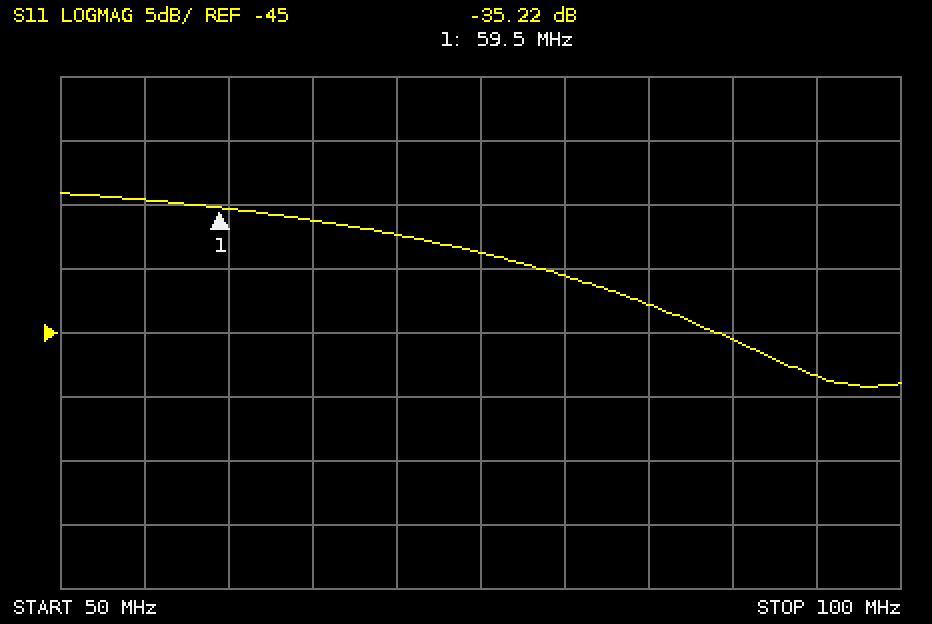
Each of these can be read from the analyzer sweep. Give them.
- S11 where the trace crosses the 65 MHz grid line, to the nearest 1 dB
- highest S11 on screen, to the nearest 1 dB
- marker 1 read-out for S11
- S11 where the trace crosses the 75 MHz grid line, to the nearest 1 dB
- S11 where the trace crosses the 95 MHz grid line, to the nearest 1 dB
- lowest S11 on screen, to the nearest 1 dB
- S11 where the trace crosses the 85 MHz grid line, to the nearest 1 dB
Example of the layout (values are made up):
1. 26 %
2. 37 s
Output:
1. -36 dB
2. -34 dB
3. -35.22 dB
4. -39 dB
5. -48 dB
6. -49 dB
7. -43 dB
